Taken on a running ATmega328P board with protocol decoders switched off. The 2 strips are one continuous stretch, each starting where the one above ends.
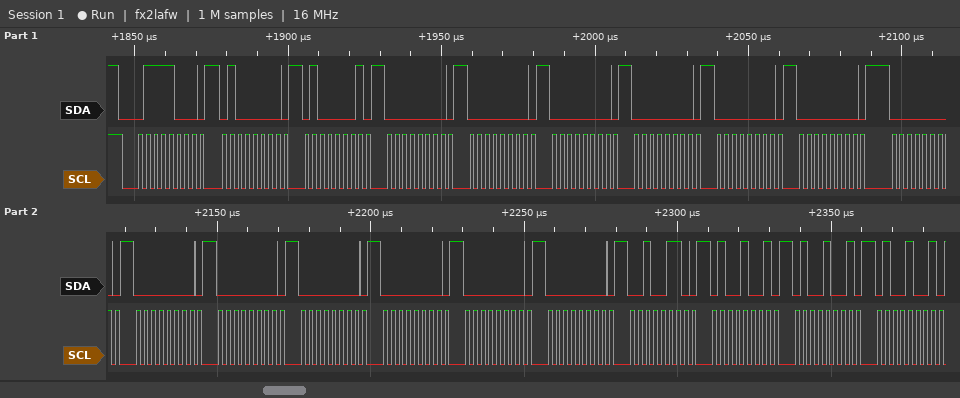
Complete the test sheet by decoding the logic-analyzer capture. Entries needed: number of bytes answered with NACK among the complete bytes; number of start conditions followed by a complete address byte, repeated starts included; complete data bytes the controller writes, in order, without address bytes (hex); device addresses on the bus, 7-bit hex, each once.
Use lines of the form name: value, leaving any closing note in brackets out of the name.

number of bytes answered with NACK among the complete bytes: 0
number of start conditions followed by a complete address byte, repeated starts included: 1
complete data bytes the controller writes, in order, without address bytes: 40 41 00 00 00 00 00 00 00 00 00 00 00 00 00 26 49 49 49
device addresses on the bus, 7-bit hex, each once: 0x3C
